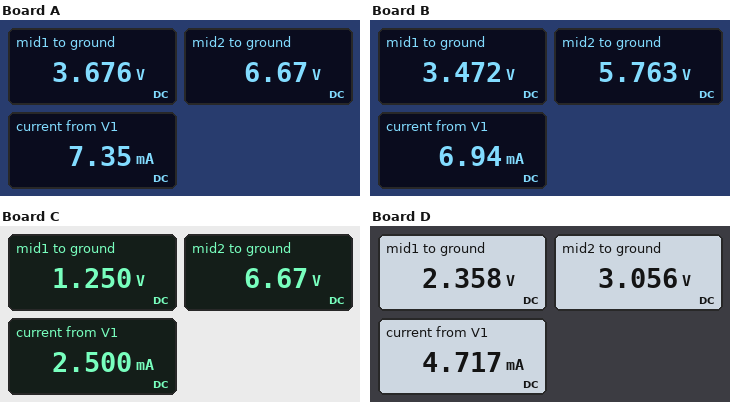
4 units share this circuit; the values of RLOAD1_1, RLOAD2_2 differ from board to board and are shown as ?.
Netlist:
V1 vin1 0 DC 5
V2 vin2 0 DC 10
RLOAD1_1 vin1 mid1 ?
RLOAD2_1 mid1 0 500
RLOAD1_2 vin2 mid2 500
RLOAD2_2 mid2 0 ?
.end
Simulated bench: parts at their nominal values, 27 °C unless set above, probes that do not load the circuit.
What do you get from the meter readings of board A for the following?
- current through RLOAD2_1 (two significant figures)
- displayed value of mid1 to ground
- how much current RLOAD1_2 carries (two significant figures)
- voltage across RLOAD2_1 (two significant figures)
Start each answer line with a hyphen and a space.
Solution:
- 7.4 mA
- 3.676 V
- 6.7 mA
- 3.7 V
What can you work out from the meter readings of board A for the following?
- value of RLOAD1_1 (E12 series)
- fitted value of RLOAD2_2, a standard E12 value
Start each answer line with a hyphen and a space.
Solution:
- 180 Ω
- 1 kΩ
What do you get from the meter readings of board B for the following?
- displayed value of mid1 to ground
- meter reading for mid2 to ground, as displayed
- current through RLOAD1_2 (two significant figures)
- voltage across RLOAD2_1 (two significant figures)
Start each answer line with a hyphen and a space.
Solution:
- 3.472 V
- 5.763 V
- 8.5 mA
- 3.5 V
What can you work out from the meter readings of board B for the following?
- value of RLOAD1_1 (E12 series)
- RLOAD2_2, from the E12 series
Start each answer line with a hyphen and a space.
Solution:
- 220 Ω
- 680 Ω
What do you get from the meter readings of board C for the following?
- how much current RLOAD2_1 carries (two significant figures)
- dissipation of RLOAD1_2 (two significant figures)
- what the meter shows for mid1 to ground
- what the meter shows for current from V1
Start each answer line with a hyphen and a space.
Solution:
- 2.5 mA
- 22 mW
- 1.250 V
- 2.500 mA
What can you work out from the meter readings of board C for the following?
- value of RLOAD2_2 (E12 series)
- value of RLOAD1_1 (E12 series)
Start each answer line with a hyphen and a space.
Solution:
- 1 kΩ
- 1.5 kΩ
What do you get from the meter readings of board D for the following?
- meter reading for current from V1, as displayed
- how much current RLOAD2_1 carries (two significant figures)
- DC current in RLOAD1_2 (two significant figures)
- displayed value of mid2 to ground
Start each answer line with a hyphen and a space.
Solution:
- 4.717 mA
- 4.7 mA
- 14 mA
- 3.056 V
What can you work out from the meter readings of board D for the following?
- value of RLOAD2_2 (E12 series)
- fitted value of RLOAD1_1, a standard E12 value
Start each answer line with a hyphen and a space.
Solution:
- 220 Ω
- 560 Ω
